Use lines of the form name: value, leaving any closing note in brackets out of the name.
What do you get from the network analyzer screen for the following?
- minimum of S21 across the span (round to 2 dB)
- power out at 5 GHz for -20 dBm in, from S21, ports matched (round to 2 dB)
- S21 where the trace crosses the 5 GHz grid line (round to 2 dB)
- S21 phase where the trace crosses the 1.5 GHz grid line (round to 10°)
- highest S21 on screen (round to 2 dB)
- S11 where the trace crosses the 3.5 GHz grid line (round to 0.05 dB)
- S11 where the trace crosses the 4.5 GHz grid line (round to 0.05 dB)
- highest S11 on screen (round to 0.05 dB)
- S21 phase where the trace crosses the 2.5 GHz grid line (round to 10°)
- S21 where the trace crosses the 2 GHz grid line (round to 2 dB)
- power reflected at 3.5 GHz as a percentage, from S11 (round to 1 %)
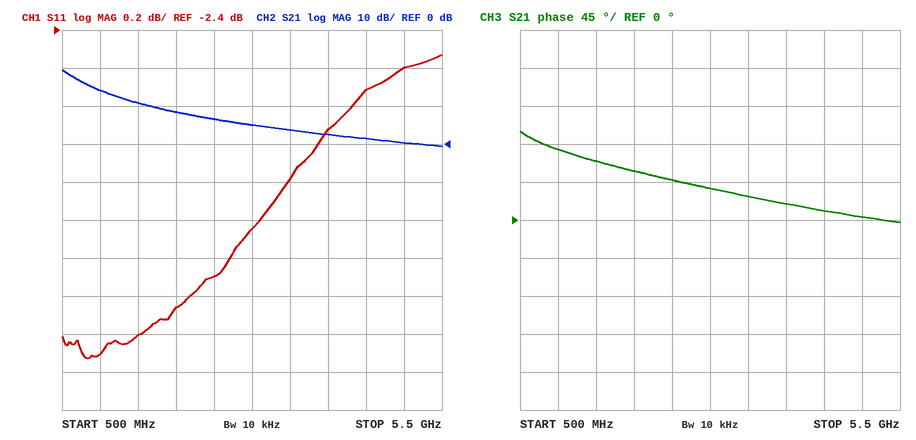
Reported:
minimum of S21 across the span: 0 dB
power out at 5 GHz for -20 dBm in, from S21, ports matched: -20 dBm
S21 where the trace crosses the 5 GHz grid line: 0 dB
S21 phase where the trace crosses the 1.5 GHz grid line: 70°
highest S21 on screen: 20 dB
S11 where the trace crosses the 3.5 GHz grid line: -3.20 dB
S11 where the trace crosses the 4.5 GHz grid line: -2.70 dB
highest S11 on screen: -2.55 dB
S21 phase where the trace crosses the 2.5 GHz grid line: 50°
S21 where the trace crosses the 2 GHz grid line: 8 dB
power reflected at 3.5 GHz as a percentage, from S11: 48 %
